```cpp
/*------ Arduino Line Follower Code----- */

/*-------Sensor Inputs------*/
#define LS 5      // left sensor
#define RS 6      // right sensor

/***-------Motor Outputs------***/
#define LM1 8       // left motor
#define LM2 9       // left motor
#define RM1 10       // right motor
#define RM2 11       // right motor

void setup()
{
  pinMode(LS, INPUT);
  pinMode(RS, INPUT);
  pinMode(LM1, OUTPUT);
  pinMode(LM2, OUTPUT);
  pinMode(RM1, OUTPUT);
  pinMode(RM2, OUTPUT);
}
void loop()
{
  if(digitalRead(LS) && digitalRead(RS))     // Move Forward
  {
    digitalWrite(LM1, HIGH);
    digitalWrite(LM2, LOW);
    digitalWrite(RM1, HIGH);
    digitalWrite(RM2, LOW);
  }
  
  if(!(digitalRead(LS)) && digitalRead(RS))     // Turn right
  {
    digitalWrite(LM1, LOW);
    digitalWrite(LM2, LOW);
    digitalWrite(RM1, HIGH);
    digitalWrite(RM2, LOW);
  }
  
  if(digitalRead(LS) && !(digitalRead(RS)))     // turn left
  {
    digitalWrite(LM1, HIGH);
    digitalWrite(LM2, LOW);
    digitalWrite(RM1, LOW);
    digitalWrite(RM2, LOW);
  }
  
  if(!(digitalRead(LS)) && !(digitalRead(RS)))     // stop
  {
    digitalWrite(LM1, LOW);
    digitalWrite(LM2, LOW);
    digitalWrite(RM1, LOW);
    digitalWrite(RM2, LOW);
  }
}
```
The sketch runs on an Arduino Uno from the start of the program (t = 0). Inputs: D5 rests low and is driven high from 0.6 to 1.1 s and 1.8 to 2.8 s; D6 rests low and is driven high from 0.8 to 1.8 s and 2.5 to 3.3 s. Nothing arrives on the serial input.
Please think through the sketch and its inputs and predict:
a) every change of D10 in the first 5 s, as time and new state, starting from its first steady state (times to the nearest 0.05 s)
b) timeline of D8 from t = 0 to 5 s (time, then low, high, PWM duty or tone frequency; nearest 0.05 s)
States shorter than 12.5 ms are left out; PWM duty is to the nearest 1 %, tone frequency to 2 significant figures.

0 s low; 0.8 s high; 1.8 s low; 2.5 s high; 3.3 s low
0 s low; 0.6 s high; 1.1 s low; 1.8 s high; 2.8 s low
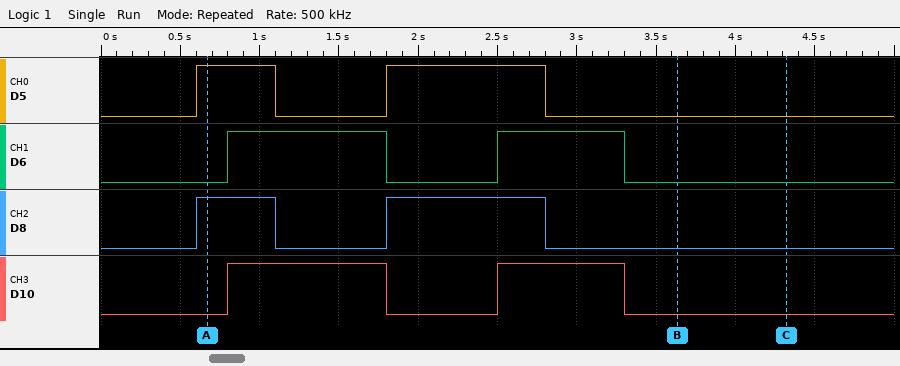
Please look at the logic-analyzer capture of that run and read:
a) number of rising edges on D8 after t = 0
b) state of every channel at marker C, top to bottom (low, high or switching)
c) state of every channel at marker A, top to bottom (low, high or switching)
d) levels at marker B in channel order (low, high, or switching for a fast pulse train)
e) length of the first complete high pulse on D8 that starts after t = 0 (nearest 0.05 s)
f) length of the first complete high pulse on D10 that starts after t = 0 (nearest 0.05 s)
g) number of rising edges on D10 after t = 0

2
D5 low, D6 low, D8 low, D10 low
D5 high, D6 low, D8 high, D10 low
D5 low, D6 low, D8 low, D10 low
0.50 s
1.00 s
2
